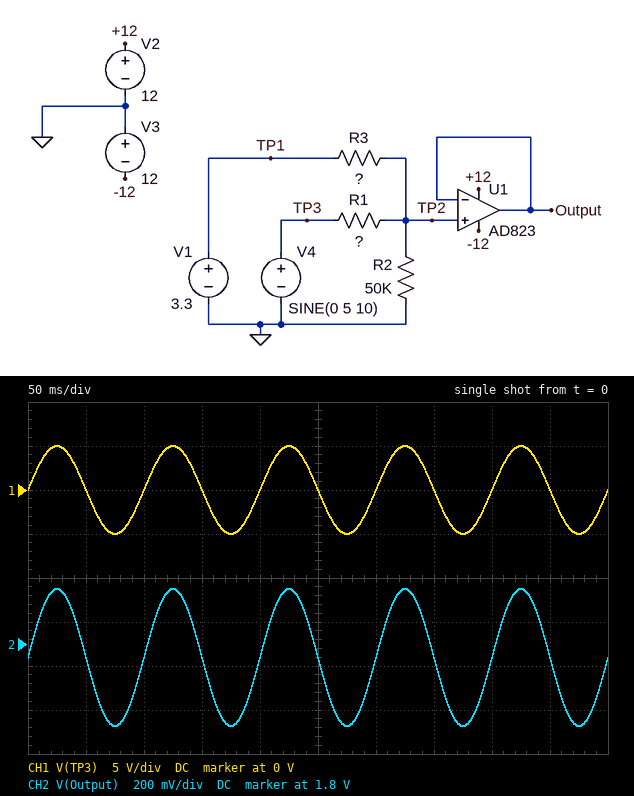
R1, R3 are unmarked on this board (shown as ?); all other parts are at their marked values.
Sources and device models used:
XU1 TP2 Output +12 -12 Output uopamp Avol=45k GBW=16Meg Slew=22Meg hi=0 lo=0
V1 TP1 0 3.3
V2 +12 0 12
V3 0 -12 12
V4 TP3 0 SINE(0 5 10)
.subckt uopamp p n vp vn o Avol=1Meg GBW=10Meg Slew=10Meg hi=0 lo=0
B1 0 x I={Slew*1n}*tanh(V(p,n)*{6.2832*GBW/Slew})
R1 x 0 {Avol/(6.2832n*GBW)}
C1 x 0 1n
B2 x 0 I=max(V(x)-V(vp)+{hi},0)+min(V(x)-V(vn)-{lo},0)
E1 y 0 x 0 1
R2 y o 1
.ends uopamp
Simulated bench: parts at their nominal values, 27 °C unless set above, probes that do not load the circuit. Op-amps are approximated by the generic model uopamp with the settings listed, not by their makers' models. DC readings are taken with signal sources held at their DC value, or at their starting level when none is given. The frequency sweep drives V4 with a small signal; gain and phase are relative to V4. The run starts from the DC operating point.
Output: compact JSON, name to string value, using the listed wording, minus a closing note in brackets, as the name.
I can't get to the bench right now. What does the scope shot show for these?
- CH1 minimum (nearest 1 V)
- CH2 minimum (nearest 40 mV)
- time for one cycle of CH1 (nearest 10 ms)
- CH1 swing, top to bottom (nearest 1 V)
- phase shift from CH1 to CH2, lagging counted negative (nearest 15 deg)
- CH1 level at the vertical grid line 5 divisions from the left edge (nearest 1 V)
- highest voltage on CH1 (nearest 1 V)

{"CH1 minimum": "-5 V", "CH2 minimum": "1.44 V", "time for one cycle of CH1": "100 ms", "CH1 swing, top to bottom": "10 V", "phase shift from CH1 to CH2, lagging counted negative": "0 deg", "CH1 level at the vertical grid line 5 divisions from the left edge": "0 V", "highest voltage on CH1": "5 V"}
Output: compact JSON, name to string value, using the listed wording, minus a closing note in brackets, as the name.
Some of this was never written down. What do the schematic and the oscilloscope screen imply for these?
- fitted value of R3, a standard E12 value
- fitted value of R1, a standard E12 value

{"fitted value of R3, a standard E12 value": "39 kΩ", "fitted value of R1, a standard E12 value": "330 kΩ"}
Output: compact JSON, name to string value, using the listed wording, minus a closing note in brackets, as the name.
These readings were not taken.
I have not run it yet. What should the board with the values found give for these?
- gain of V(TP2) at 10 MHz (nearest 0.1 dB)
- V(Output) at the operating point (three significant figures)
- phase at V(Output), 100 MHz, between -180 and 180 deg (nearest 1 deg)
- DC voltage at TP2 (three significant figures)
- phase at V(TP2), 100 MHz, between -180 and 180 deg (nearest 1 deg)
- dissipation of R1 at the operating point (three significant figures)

{"gain of V(TP2) at 10 MHz": "-24.1 dB", "V(Output) at the operating point": "1.74 V", "phase at V(Output), 100 MHz, between -180 and 180 deg": "-81 deg", "DC voltage at TP2": "1.74 V", "phase at V(TP2), 100 MHz, between -180 and 180 deg": "0 deg", "dissipation of R1 at the operating point": "9.16 µW"}
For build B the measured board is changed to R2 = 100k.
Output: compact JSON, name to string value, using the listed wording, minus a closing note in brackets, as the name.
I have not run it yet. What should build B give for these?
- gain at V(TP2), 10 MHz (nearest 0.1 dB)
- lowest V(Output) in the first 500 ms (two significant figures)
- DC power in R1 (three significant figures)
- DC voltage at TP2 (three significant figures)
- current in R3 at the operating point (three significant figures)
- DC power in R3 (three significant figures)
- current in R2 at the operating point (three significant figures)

{"gain at V(TP2), 10 MHz": "-22.1 dB", "lowest V(Output) in the first 500 ms": "1.8 V", "DC power in R1": "14.5 µW", "DC voltage at TP2": "2.19 V", "current in R3 at the operating point": "28.5 µA", "DC power in R3": "31.7 µW", "current in R2 at the operating point": "21.9 µA"}
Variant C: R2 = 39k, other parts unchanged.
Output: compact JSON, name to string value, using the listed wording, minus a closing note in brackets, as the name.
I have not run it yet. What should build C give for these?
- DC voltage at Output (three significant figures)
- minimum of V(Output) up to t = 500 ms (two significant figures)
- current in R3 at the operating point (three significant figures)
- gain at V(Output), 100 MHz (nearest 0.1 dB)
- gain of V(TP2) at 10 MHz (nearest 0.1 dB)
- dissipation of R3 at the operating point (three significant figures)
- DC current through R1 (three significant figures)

{"DC voltage at Output": "1.56 V", "minimum of V(Output) up to t = 500 ms": "1.3 V", "current in R3 at the operating point": "44.7 µA", "gain at V(Output), 100 MHz": "-41.1 dB", "gain of V(TP2) at 10 MHz": "-25.1 dB", "dissipation of R3 at the operating point": "77.8 µW", "DC current through R1": "4.72 µA"}
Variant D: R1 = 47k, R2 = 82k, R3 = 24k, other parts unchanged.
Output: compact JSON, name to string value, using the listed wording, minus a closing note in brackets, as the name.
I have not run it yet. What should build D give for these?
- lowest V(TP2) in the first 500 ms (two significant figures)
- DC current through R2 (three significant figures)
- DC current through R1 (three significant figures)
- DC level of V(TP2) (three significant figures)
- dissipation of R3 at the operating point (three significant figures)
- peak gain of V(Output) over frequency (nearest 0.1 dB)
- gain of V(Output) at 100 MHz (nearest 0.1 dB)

{"lowest V(TP2) in the first 500 ms": "410 mV", "DC current through R2": "22.3 µA", "DC current through R1": "38.9 µA", "DC level of V(TP2)": "1.83 V", "dissipation of R3 at the operating point": "90.0 µW", "peak gain of V(Output) over frequency": "-11.0 dB", "gain of V(Output) at 100 MHz": "-27.0 dB"}
